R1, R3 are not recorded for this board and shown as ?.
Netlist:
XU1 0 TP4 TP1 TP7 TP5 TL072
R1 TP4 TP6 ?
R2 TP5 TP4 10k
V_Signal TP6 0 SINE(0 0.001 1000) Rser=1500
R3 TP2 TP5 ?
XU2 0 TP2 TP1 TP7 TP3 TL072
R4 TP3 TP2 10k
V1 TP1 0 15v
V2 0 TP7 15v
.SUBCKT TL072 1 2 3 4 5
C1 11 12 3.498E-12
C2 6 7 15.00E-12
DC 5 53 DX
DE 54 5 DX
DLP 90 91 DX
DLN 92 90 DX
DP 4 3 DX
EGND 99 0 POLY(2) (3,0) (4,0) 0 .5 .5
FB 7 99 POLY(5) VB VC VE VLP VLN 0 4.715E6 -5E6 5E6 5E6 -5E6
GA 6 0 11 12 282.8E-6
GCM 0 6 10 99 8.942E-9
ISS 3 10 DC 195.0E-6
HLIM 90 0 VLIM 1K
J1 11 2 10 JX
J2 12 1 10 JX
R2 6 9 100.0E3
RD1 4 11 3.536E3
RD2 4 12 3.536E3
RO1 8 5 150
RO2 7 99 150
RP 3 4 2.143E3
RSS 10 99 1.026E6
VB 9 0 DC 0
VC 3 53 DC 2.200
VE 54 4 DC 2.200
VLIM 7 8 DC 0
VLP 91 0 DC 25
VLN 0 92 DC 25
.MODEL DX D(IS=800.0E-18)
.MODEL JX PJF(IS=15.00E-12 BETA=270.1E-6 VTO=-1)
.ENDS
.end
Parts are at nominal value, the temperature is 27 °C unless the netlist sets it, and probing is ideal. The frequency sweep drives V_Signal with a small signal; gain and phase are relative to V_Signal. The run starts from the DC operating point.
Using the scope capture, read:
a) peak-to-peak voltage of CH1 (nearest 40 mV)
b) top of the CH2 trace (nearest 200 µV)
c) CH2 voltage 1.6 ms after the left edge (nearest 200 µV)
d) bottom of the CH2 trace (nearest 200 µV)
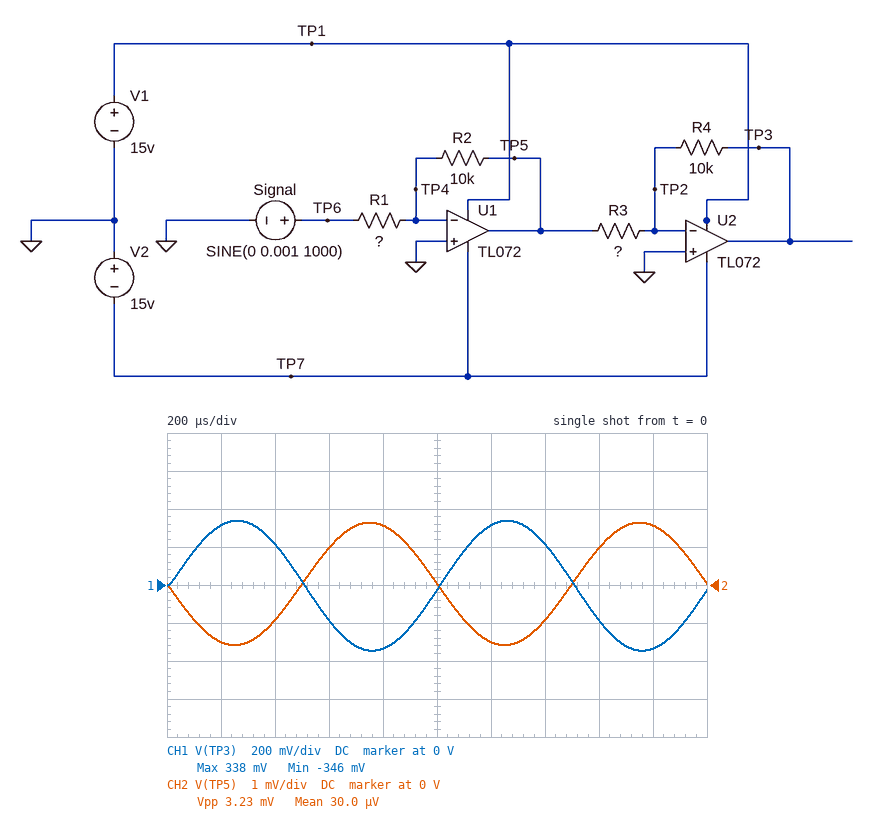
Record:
680 mV
1.6 mV
1.0 mV
-1.6 mV
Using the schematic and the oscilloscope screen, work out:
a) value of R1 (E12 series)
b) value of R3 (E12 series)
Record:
4.7 kΩ
47 Ω
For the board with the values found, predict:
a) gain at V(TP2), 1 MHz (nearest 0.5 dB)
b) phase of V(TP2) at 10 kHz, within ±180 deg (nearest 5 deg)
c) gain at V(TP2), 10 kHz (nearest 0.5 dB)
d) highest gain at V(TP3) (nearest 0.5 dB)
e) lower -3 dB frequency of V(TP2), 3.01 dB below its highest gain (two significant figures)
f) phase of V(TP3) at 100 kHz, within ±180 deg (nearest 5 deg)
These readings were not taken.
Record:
2.5 dB
-125 deg
-1.5 dB
50.5 dB
15 kHz
-85 deg
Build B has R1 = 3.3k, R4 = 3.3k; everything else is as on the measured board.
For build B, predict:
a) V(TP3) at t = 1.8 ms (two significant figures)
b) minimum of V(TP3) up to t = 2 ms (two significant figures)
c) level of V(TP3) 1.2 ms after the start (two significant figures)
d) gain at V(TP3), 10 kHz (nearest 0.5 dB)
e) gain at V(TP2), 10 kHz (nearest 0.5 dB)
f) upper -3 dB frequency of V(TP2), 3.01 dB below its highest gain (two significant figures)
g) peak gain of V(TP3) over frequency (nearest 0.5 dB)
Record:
-140 mV
-150 mV
140 mV
43.0 dB
-7.5 dB
1.5 MHz
43.5 dB
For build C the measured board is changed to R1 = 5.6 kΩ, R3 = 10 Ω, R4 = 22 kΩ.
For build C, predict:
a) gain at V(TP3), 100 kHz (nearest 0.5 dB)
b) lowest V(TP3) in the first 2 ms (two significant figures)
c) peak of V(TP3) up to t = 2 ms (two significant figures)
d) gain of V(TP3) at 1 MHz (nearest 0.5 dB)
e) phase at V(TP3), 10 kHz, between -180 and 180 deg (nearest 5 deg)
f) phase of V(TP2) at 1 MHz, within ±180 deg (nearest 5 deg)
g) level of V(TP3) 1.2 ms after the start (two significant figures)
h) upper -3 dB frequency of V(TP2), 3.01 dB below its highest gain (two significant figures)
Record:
33.5 dB
-2.6 V
2.6 V
12.5 dB
-80 deg
140 deg
1.6 V
1.8 MHz
